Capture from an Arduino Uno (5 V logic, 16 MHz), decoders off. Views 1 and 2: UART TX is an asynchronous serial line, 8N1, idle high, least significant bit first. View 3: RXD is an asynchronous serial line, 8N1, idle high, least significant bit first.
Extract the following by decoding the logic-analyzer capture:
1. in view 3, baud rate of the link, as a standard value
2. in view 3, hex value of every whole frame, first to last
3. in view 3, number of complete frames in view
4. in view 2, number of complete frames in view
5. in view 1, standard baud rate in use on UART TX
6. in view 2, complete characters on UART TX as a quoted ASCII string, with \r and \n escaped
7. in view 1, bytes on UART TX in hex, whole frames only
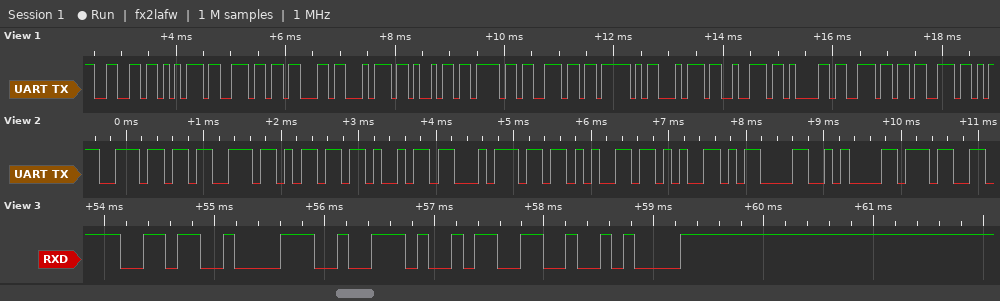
9600 baud
36 38 2E 33 0A
5
10
9600 baud
"nsmit++\r\n7"
66 75 6E 63 74 69 6F 6E 5F 74 72 61 6E 73
